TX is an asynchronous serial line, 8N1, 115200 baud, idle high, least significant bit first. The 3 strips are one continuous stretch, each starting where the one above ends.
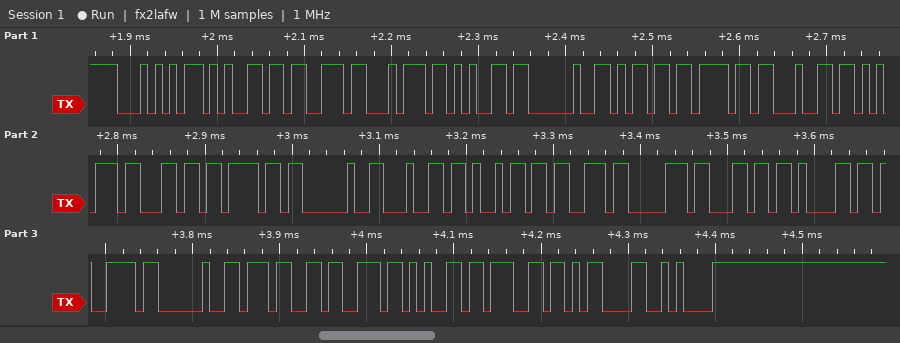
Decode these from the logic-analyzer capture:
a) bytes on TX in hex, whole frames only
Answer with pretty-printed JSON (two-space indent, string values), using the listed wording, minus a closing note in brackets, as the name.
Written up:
{
  "bytes on TX in hex, whole frames only": "0x54 0x65 0x73 0x74 0x65 0x20 0x6D 0x6F 0x64 0x75 0x6C 0x6F 0x20 0x64 0x69 0x73 0x70 0x6C 0x61 0x79 0x20 0x37 0x73 0x65 0x67 0x0D 0x0A"
}
